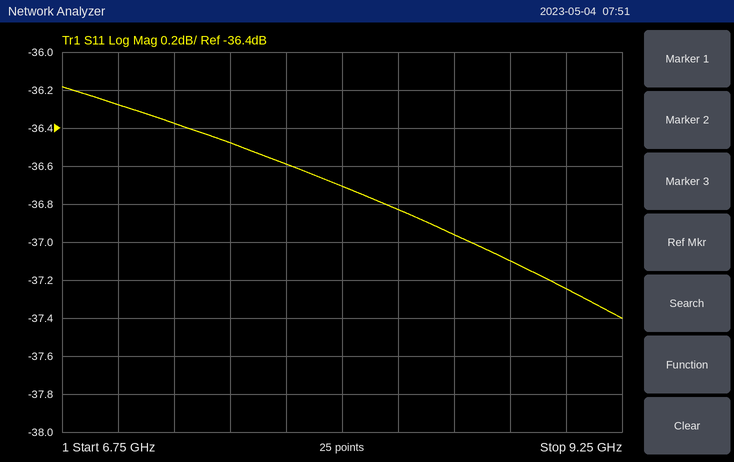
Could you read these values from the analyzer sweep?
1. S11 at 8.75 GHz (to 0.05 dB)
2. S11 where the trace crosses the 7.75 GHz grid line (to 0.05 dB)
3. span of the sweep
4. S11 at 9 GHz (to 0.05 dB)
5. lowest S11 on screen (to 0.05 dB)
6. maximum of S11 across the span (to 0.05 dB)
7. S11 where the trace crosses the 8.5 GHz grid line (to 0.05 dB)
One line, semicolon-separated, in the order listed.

-37.10 dB; -36.60 dB; 2.5 GHz; -37.25 dB; -37.40 dB; -36.20 dB; -36.95 dB
